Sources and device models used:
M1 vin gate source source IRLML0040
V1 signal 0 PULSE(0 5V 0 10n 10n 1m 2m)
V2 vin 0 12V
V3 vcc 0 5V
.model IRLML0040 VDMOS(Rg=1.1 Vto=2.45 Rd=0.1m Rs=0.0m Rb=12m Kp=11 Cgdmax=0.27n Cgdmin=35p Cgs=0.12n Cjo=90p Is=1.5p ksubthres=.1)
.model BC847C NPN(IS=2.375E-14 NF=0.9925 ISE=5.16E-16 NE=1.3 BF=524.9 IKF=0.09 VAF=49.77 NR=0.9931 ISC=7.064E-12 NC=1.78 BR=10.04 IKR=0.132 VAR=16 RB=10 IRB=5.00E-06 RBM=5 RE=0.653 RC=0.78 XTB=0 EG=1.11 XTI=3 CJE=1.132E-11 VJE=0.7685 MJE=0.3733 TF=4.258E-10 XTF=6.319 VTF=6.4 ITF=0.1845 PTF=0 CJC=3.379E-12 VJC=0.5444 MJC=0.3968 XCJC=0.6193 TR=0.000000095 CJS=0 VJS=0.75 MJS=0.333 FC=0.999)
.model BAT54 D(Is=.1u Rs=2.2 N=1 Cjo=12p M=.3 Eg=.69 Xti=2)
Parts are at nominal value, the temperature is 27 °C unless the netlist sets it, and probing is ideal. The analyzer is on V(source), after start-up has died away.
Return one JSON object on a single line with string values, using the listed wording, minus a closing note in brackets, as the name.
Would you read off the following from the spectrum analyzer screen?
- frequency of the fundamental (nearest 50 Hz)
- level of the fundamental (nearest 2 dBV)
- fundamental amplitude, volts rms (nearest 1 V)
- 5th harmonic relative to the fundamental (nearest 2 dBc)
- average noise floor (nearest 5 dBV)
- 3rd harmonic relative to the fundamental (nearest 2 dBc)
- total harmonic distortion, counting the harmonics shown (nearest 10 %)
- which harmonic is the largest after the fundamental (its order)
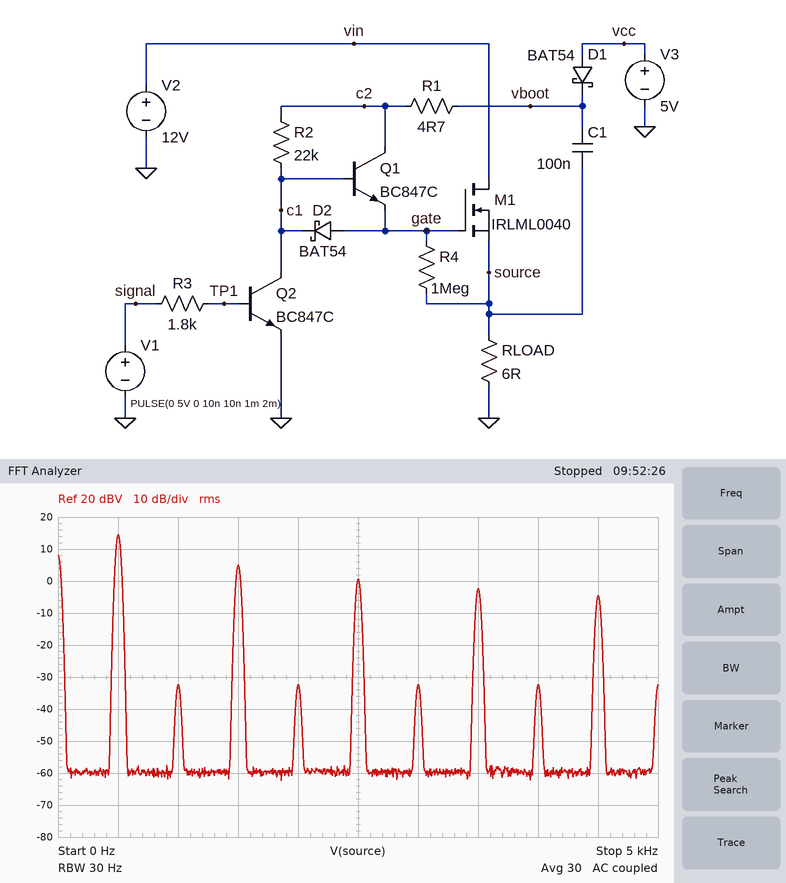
{"frequency of the fundamental": "500 Hz", "level of the fundamental": "14 dBV", "fundamental amplitude, volts rms": "5 V", "5th harmonic relative to the fundamental": "-14 dBc", "average noise floor": "-60 dBV", "3rd harmonic relative to the fundamental": "-10 dBc", "total harmonic distortion, counting the harmonics shown": "40 %", "which harmonic is the largest after the fundamental": "3"}
